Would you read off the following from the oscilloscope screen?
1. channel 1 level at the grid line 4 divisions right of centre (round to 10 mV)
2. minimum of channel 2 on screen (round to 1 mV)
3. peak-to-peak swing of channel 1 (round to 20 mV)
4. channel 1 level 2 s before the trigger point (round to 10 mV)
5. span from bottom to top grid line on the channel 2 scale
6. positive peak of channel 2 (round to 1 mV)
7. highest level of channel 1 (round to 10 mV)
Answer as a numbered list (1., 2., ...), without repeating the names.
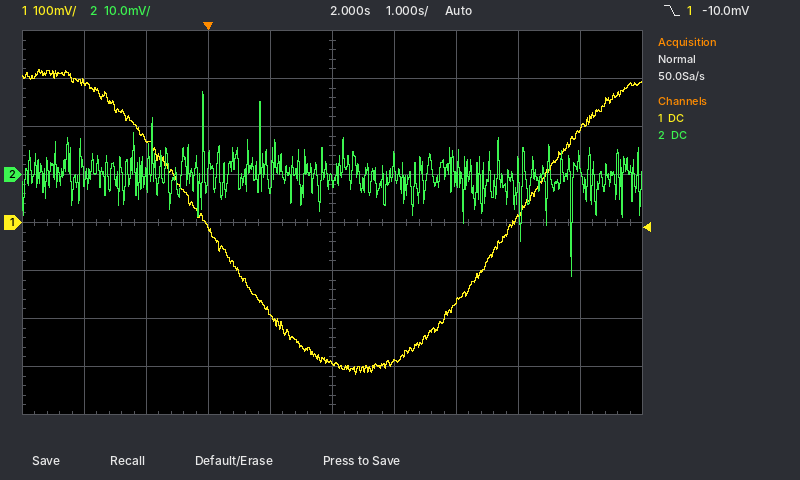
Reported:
1. 200 mV
2. -21 mV
3. 640 mV
4. 290 mV
5. 80 mV
6. 17 mV
7. 320 mV
